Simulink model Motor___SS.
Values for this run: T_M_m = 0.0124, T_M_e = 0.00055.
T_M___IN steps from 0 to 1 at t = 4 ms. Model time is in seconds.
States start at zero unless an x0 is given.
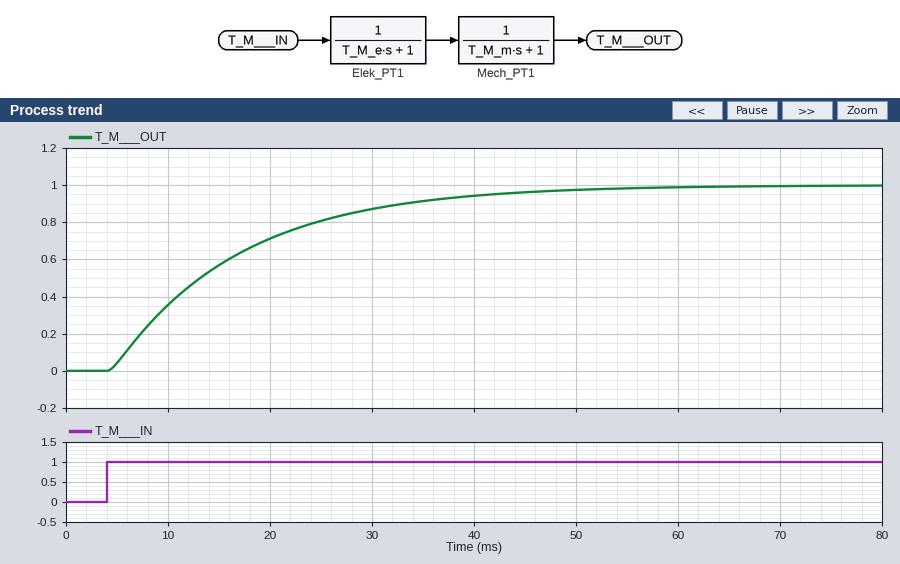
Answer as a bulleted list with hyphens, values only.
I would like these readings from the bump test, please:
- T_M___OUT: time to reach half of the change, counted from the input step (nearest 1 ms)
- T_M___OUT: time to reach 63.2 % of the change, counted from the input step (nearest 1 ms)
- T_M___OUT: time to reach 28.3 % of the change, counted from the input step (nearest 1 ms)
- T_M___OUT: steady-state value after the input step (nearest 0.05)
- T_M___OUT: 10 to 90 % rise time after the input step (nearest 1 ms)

- 9 ms
- 13 ms
- 5 ms
- 1.00
- 27 ms
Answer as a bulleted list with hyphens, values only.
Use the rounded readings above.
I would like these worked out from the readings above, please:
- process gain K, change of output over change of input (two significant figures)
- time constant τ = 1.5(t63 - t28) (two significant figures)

- 1.0
- 12 ms
